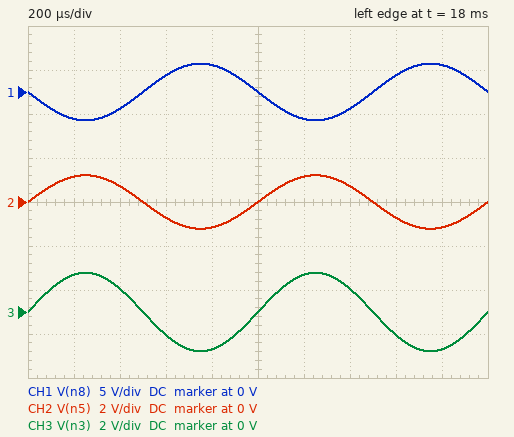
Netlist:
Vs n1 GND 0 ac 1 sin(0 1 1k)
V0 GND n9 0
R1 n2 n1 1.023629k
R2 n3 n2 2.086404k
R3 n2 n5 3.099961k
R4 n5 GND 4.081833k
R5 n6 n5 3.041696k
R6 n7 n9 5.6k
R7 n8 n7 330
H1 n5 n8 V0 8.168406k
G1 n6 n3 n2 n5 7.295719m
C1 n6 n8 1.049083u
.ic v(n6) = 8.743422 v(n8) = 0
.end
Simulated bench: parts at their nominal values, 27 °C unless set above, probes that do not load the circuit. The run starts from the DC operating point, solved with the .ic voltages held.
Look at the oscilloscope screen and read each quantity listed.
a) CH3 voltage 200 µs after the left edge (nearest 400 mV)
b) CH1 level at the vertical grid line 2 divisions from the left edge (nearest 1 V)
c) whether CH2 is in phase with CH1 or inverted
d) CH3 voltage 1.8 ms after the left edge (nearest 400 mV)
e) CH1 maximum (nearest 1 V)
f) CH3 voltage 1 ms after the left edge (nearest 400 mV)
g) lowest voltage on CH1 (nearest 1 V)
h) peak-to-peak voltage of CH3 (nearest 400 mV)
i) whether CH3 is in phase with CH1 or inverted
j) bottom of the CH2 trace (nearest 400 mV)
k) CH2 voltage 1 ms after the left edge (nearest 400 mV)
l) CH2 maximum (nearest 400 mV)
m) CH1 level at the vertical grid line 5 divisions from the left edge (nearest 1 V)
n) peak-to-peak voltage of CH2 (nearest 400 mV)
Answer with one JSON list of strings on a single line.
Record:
["1.6 V", "-2 V", "inverted", "-1.6 V", "3 V", "0 V", "-3 V", "3.6 V", "inverted", "-1.2 V", "0 V", "1.2 V", "0 V", "2.4 V"]
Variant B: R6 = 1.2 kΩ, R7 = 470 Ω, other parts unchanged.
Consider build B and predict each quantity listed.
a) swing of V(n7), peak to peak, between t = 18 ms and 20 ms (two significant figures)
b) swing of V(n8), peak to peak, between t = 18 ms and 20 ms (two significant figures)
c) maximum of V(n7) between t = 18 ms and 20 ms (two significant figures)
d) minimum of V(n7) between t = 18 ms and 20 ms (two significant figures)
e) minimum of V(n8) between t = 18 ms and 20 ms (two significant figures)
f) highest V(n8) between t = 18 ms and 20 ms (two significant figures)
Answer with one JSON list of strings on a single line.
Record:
["340 mV", "480 mV", "170 mV", "-170 mV", "-240 mV", "240 mV"]
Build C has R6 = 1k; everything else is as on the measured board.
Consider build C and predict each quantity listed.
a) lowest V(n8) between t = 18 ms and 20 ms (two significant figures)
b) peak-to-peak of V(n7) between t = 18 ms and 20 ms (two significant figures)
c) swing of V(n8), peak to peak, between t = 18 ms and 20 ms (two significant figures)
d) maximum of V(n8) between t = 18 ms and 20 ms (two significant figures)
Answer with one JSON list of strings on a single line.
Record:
["-180 mV", "270 mV", "360 mV", "180 mV"]
